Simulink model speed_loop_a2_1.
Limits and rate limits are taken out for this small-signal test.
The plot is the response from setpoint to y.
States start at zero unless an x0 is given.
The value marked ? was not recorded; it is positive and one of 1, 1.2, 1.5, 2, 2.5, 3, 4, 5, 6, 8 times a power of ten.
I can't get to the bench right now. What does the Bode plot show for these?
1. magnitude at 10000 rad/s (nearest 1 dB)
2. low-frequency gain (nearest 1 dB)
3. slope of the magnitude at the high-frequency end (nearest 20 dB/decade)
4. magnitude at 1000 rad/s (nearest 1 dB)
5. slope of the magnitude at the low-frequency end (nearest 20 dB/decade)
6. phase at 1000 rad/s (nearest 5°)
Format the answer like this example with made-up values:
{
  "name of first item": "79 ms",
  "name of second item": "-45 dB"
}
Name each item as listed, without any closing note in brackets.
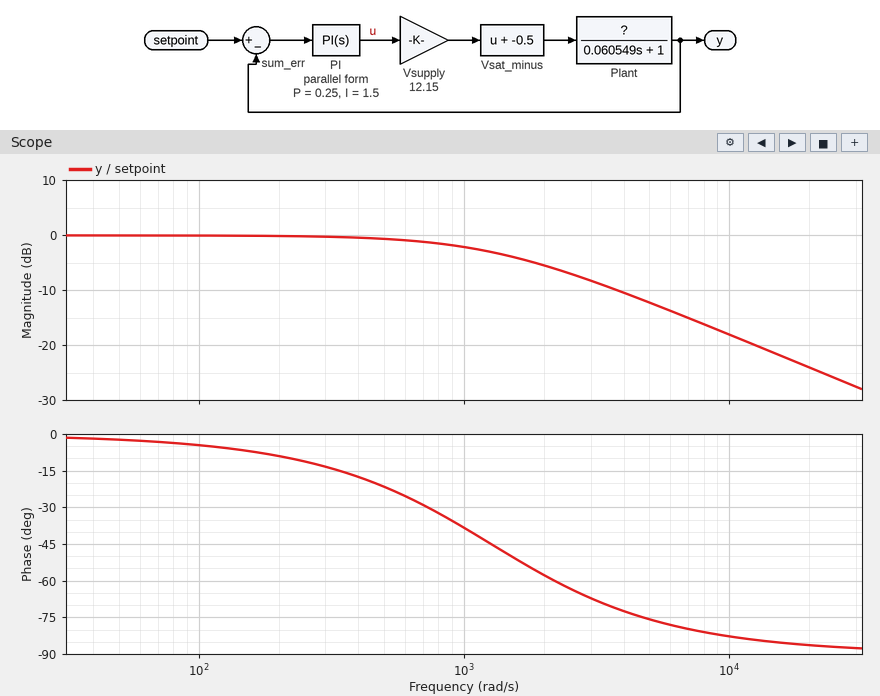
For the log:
{
  "magnitude at 10000 rad/s": "-18 dB",
  "low-frequency gain": "0 dB",
  "slope of the magnitude at the high-frequency end": "-20 dB/decade",
  "magnitude at 1000 rad/s": "-2 dB",
  "slope of the magnitude at the low-frequency end": "0 dB/decade",
  "phase at 1000 rad/s": "-40°"
}
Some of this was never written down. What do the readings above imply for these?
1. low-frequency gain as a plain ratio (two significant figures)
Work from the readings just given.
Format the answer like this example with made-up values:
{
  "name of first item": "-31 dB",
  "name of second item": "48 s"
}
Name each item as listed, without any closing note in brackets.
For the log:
{
  "low-frequency gain as a plain ratio": "1.0"
}
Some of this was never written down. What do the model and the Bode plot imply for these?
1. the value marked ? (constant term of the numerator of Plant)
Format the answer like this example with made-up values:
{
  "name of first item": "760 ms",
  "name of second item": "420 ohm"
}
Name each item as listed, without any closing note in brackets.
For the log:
{
  "the value marked ?": "25"
}
